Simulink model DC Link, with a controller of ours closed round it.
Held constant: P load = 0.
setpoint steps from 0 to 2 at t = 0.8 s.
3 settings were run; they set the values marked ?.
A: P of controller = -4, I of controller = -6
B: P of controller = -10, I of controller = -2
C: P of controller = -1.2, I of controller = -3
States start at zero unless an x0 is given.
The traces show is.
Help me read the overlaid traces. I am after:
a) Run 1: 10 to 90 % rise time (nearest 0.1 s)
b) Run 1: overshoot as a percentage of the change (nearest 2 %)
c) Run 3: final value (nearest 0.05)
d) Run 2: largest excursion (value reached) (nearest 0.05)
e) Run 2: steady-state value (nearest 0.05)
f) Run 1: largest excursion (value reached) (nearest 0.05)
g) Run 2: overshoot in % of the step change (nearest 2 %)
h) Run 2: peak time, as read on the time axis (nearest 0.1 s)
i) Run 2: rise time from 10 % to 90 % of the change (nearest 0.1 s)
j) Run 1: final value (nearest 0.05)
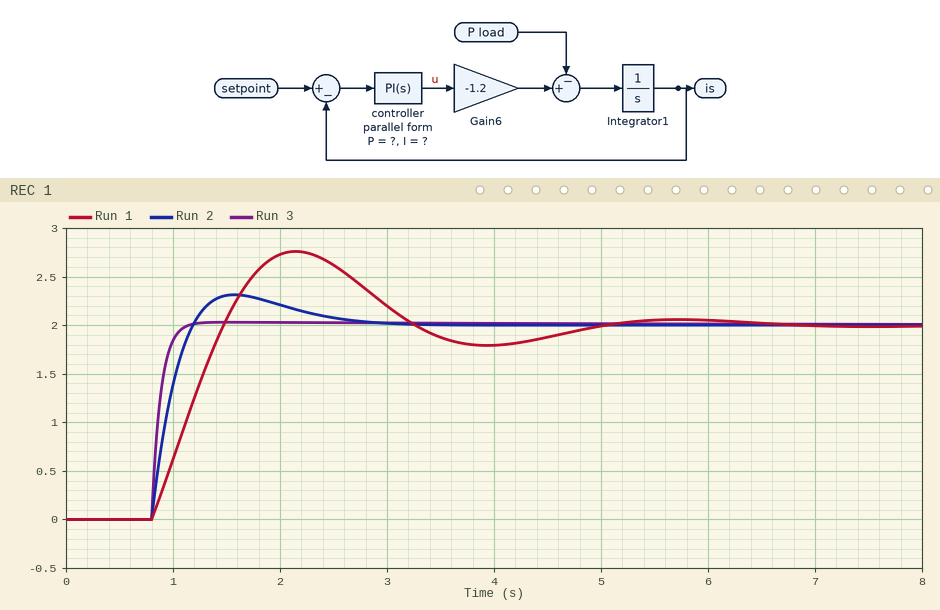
0.5 s
38 %
2.00
2.30
2.00
2.75
16 %
1.6 s
0.3 s
2.00
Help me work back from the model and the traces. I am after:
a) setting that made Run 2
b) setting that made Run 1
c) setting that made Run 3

A
C
B
